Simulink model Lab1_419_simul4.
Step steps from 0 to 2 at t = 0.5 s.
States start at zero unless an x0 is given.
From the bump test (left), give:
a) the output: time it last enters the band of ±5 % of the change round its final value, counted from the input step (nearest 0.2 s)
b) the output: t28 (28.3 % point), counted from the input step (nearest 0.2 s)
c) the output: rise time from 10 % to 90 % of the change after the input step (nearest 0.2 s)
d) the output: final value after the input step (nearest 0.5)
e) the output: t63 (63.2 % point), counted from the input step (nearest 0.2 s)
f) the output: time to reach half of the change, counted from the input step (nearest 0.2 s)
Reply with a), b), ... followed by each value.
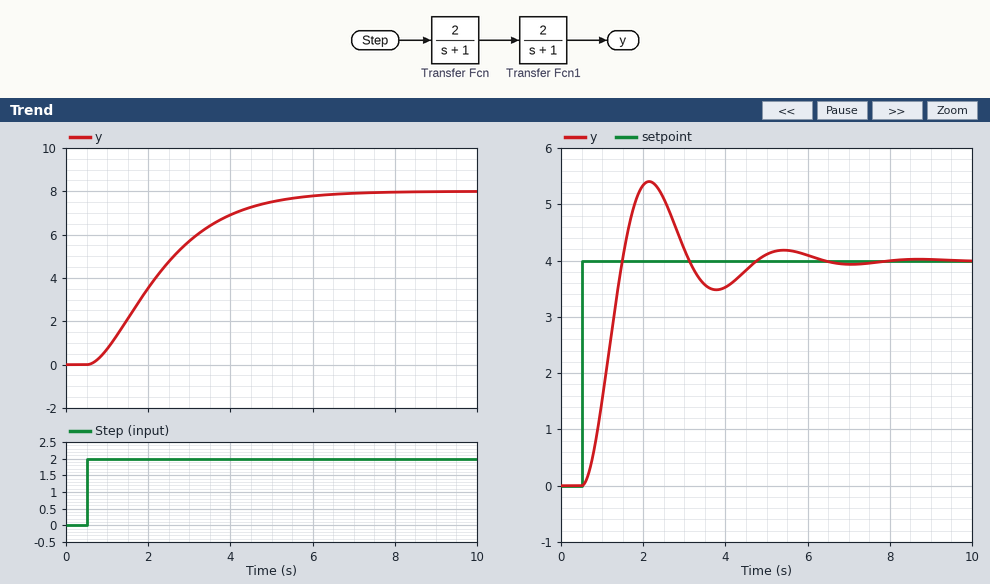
a) 4.8 s
b) 1.0 s
c) 3.4 s
d) 8.0
e) 2.2 s
f) 1.6 s
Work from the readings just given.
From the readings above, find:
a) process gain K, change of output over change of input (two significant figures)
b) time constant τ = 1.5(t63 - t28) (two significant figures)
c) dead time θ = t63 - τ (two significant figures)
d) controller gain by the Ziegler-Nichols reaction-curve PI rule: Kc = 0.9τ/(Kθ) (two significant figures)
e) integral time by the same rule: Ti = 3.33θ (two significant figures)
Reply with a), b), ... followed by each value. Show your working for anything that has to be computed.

a) (8 - 0) / 2 = 4.0
b) 1.5 × (2.2 - 1) = 1.8 s
c) 2.2 - 1.8 = 0.40 s
d) 0.9 × 1.8 / (4 × 0.4) = 1.0
e) 3.33 × 0.4 = 1.3 s
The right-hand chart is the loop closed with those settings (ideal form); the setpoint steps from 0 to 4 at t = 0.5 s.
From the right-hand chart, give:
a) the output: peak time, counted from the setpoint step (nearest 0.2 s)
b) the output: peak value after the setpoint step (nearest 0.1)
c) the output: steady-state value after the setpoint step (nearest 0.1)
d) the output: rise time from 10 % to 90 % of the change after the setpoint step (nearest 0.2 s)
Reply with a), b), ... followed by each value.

a) 1.6 s
b) 5.4
c) 4.0
d) 0.6 s
